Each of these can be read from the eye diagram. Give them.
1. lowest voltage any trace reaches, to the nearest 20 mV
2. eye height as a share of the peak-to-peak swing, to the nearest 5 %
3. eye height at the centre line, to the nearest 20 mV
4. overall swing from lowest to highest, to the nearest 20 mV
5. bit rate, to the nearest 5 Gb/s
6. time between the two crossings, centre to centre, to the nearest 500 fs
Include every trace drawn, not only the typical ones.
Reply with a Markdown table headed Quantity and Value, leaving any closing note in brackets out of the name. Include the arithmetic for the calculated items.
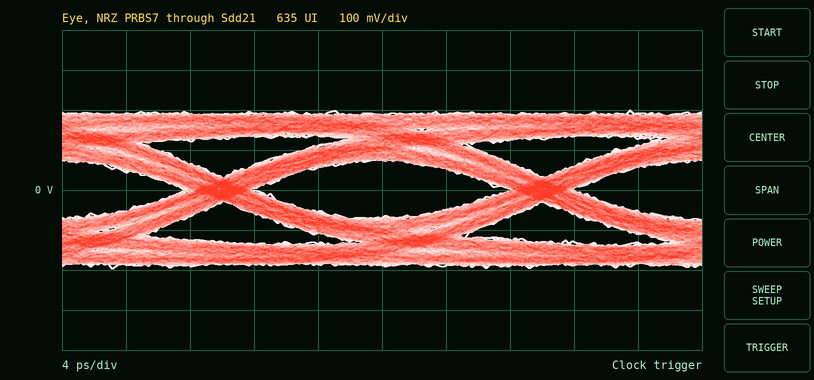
| Quantity | Value |
|---|---|
| lowest voltage any trace reaches, to the nearest 20 mV | -200 mV |
| eye height as a share of the peak-to-peak swing, to the nearest 5 % | 140 mV / 400 mV ≈ 35 % |
| eye height at the centre line, to the nearest 20 mV | 140 mV |
| overall swing from lowest to highest, to the nearest 20 mV | 400 mV |
| bit rate, to the nearest 5 Gb/s | 50 Gb/s |
| time between the two crossings, centre to centre, to the nearest 500 fs | 20.0 ps |
